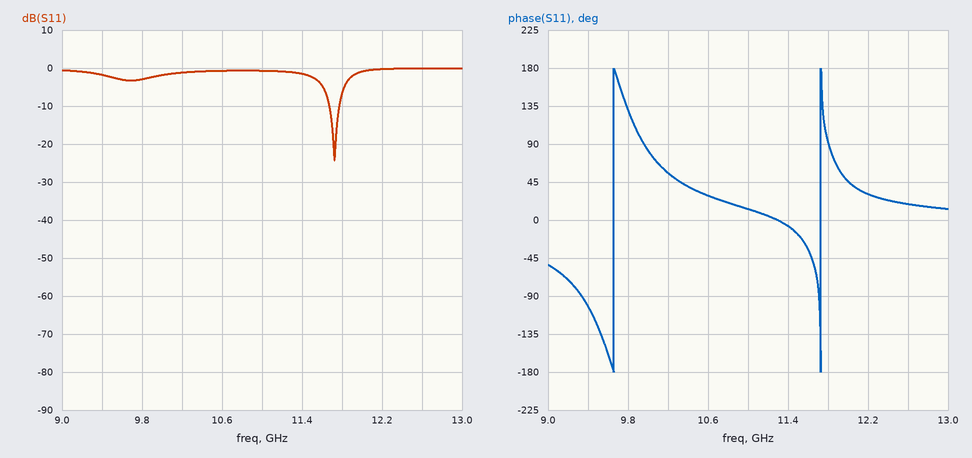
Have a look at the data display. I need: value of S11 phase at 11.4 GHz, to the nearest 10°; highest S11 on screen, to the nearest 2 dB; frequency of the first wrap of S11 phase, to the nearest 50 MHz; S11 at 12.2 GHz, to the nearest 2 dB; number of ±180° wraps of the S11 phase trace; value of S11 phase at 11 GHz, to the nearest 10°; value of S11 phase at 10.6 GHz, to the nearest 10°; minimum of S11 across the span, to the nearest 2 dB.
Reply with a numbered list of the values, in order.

1. -10°
2. 0 dB
3. 9.65 GHz
4. 0 dB
5. 2
6. 10°
7. 30°
8. -24 dB
